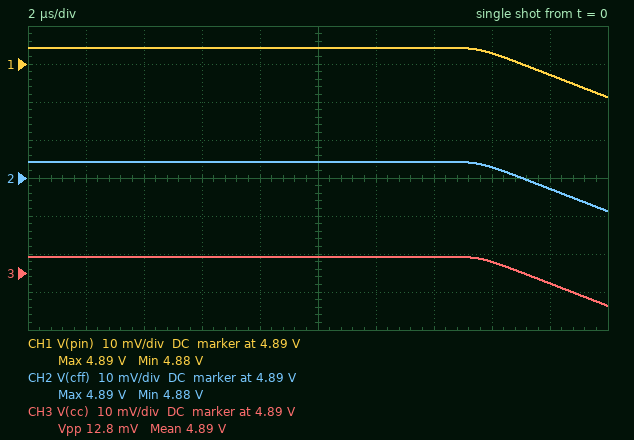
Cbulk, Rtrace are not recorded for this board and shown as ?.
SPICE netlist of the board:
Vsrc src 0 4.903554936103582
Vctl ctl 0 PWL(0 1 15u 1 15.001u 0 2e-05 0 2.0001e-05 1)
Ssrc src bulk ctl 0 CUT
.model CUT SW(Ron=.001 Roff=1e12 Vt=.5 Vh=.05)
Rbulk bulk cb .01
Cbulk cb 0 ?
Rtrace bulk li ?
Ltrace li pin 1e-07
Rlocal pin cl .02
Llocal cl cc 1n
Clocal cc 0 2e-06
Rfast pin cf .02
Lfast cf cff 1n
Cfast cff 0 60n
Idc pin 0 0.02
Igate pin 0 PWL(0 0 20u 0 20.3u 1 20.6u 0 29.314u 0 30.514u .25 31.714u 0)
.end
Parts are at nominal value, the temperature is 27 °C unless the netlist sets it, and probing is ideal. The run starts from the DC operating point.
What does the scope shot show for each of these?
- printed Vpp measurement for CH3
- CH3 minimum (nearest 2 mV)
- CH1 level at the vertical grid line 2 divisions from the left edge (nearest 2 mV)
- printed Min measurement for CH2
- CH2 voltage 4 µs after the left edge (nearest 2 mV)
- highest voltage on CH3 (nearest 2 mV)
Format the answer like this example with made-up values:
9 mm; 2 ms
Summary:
12.8 mV; 4.882 V; 4.894 V; 4.88 V; 4.894 V; 4.894 V
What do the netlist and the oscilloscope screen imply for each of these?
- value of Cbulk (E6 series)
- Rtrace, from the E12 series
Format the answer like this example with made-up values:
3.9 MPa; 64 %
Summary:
4.7 µF; 0.47 Ω
